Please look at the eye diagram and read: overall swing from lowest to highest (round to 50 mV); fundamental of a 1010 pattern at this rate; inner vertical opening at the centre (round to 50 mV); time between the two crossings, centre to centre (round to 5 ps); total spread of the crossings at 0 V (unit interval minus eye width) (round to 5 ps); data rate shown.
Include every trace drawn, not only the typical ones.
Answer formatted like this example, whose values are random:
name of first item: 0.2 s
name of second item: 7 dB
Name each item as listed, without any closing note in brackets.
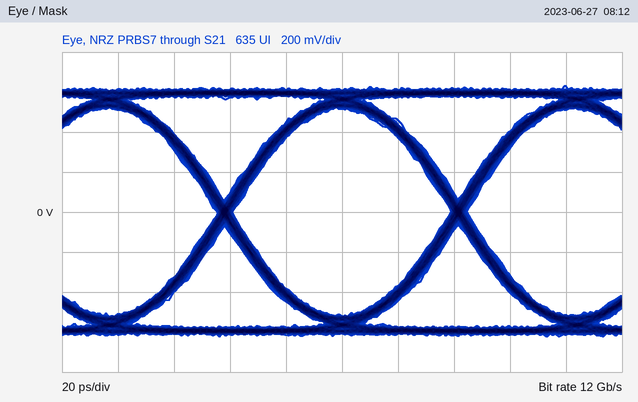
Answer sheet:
overall swing from lowest to highest: 1.25 V
fundamental of a 1010 pattern at this rate: 6 GHz
inner vertical opening at the centre: 1.05 V
time between the two crossings, centre to centre: 85 ps
total spread of the crossings at 0 V (unit interval minus eye width): 5 ps
data rate shown: 12 Gb/s
